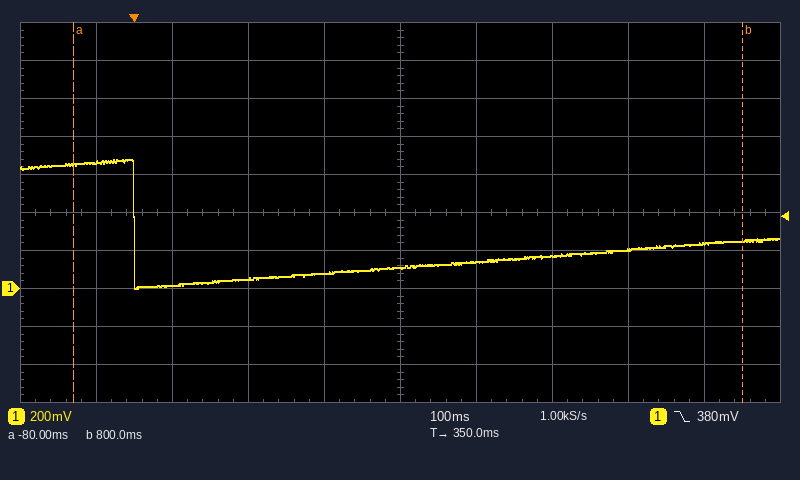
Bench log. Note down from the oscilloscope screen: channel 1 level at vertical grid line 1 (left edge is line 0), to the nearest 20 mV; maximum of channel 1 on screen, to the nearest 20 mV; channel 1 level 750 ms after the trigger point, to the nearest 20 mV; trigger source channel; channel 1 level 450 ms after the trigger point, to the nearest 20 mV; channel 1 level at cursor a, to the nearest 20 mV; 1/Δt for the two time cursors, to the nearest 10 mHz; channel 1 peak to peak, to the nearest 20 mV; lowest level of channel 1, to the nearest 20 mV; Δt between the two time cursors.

660 mV
680 mV
240 mV
channel 1
140 mV
660 mV
1.14 Hz
680 mV
0 mV
880 ms
